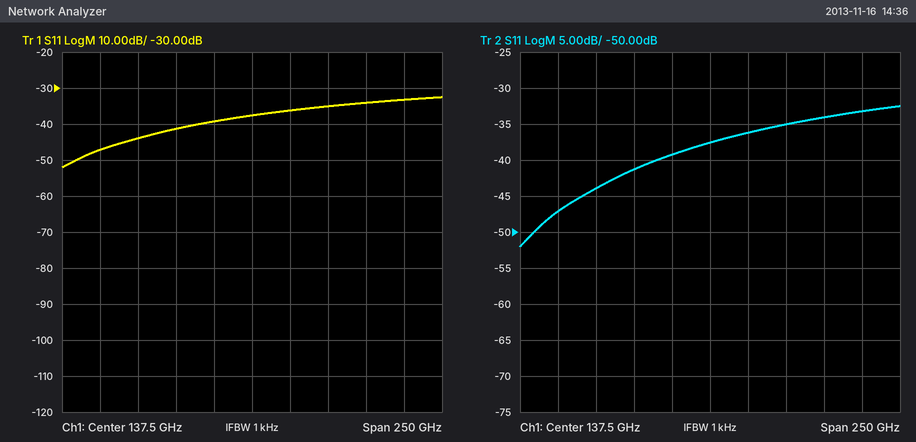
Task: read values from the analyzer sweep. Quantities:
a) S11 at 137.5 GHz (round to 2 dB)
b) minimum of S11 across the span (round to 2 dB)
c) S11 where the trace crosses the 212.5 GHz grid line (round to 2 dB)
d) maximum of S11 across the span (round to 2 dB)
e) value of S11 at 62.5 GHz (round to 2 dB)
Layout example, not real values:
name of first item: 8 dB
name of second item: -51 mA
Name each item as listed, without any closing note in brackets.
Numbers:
S11 at 137.5 GHz: -38 dB
minimum of S11 across the span: -52 dB
S11 where the trace crosses the 212.5 GHz grid line: -34 dB
maximum of S11 across the span: -32 dB
value of S11 at 62.5 GHz: -44 dB
